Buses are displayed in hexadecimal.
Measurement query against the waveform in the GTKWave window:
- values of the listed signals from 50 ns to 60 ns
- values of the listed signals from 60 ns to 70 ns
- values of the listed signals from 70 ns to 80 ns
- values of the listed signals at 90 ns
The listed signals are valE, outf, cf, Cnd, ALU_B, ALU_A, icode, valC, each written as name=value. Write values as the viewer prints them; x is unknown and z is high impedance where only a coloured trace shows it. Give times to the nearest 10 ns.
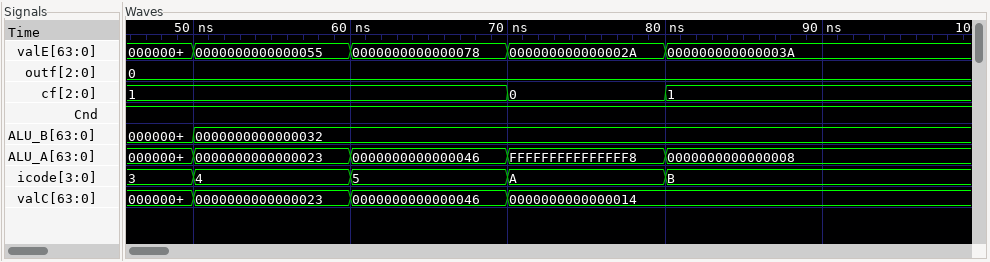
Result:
valE=0000000000000055, outf=0, cf=1, Cnd=1, ALU_B=0000000000000032, ALU_A=0000000000000023, icode=4, valC=0000000000000023
valE=0000000000000078, outf=0, cf=1, Cnd=1, ALU_B=0000000000000032, ALU_A=0000000000000046, icode=5, valC=0000000000000046
valE=000000000000002A, outf=0, cf=0, Cnd=1, ALU_B=0000000000000032, ALU_A=FFFFFFFFFFFFFFF8, icode=A, valC=0000000000000014
valE=000000000000003A, outf=0, cf=1, Cnd=1, ALU_B=0000000000000032, ALU_A=0000000000000008, icode=B, valC=0000000000000014
